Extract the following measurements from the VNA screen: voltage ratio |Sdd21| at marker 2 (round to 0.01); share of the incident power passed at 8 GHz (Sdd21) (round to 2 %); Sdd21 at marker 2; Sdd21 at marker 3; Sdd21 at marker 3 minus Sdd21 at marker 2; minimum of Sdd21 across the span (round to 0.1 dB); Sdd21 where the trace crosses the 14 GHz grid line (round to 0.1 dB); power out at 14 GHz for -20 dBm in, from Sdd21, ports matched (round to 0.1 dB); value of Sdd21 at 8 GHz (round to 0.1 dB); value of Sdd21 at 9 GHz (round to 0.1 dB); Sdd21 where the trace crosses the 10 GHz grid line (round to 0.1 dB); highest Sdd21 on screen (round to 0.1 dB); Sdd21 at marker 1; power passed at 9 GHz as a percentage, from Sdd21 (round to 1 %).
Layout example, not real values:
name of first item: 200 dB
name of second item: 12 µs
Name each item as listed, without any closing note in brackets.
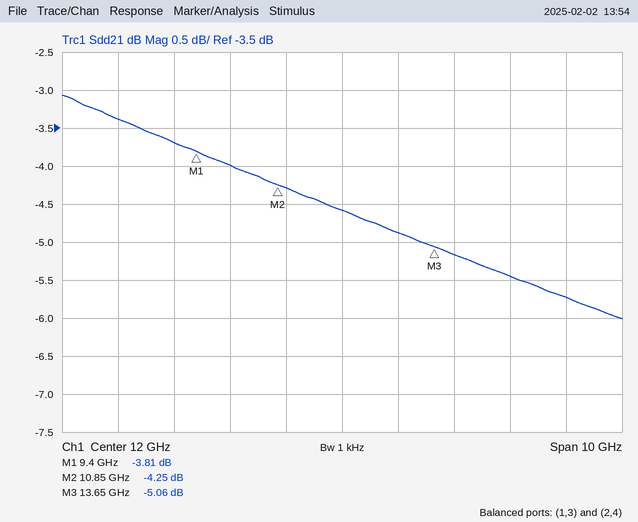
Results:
voltage ratio |Sdd21| at marker 2: 0.61
share of the incident power passed at 8 GHz (Sdd21): 46 %
Sdd21 at marker 2: -4.25 dB
Sdd21 at marker 3: -5.06 dB
Sdd21 at marker 3 minus Sdd21 at marker 2: -0.81 dB
minimum of Sdd21 across the span: -6.0 dB
Sdd21 where the trace crosses the 14 GHz grid line: -5.2 dB
power out at 14 GHz for -20 dBm in, from Sdd21, ports matched: -25.2 dBm
value of Sdd21 at 8 GHz: -3.4 dB
value of Sdd21 at 9 GHz: -3.7 dB
Sdd21 where the trace crosses the 10 GHz grid line: -4.0 dB
highest Sdd21 on screen: -3.1 dB
Sdd21 at marker 1: -3.81 dB
power passed at 9 GHz as a percentage, from Sdd21: 43 %
